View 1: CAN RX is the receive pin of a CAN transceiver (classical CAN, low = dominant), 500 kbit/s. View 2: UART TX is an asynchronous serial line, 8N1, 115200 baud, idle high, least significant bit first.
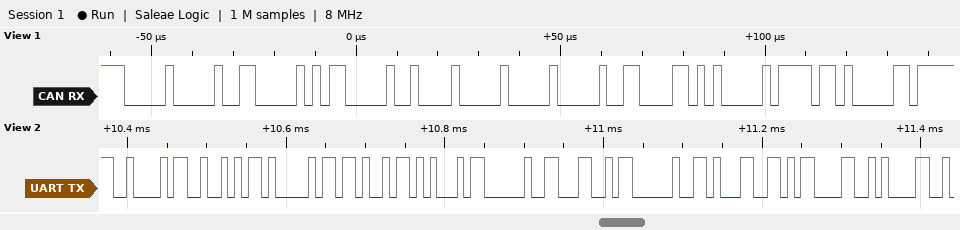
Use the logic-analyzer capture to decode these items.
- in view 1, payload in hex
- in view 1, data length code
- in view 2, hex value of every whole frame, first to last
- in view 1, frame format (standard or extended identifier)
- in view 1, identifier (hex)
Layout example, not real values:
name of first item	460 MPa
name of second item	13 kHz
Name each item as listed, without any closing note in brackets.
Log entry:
in view 1, payload in hex	00 01 86 A0
in view 1, data length code	4
in view 2, hex value of every whole frame, first to last	0x42 0x52 0x41 0x4B 0x45 0x20 0x4C 0x20 0x31 0x0D 0x0A
in view 1, frame format	extended
in view 1, identifier	0x00000B01
